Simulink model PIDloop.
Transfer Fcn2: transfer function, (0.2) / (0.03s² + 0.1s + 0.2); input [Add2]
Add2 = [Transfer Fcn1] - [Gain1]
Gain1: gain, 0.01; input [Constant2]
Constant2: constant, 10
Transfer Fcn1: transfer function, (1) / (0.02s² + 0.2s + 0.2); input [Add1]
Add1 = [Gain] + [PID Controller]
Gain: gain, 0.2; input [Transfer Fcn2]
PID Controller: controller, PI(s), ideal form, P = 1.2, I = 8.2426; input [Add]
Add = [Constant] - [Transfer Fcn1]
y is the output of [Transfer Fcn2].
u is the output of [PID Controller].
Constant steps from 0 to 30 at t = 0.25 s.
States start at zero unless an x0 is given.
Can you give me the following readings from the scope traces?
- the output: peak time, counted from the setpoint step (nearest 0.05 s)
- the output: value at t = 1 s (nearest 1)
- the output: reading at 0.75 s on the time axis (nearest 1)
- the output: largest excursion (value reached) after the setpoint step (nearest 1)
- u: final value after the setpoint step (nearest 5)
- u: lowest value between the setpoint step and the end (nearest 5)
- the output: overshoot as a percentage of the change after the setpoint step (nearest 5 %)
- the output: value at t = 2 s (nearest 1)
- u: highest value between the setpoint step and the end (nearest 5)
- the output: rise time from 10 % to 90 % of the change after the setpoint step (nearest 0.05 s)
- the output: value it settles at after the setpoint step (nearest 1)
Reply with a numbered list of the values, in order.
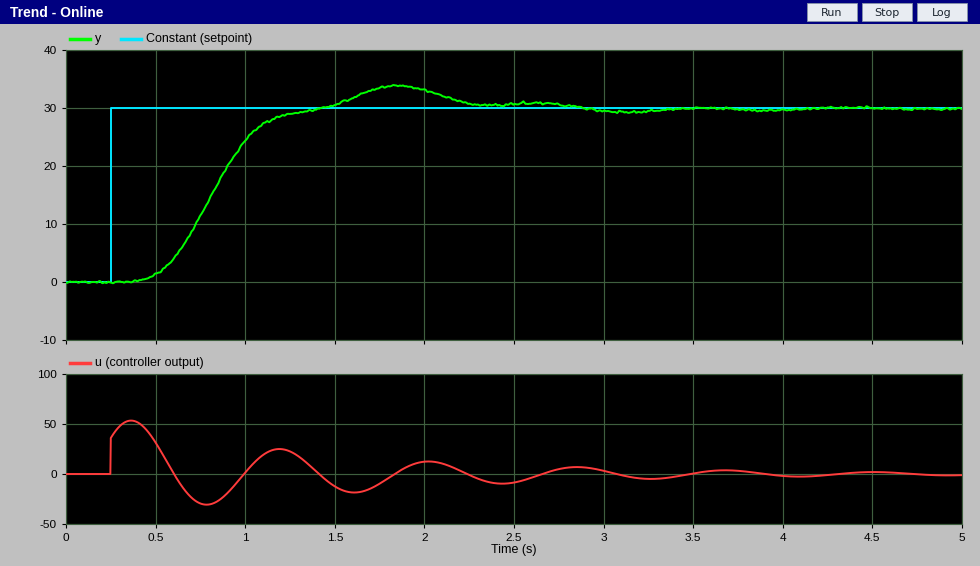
1. 1.60 s
2. 24
3. 11
4. 34
5. 0
6. -30
7. 15 %
8. 33
9. 55
10. 0.50 s
11. 30
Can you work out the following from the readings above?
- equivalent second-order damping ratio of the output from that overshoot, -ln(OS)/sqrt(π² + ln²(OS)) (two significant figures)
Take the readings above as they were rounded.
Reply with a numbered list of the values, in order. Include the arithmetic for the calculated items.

1. ln(0.15) = -1.897; 1.897 / sqrt(9.870 + 3.599) = 0.52
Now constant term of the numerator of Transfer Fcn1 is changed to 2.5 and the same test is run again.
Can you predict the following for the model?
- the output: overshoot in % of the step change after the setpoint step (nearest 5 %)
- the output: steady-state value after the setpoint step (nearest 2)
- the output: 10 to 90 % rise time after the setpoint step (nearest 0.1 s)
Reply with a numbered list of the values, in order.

1. 10 %
2. 30
3. 0.7 s
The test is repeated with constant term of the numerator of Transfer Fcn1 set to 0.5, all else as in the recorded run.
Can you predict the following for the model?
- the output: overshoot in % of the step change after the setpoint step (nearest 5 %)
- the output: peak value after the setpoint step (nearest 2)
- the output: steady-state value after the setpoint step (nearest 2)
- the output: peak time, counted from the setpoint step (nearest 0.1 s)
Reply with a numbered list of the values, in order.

1. 20 %
2. 36
3. 30
4. 1.2 s
